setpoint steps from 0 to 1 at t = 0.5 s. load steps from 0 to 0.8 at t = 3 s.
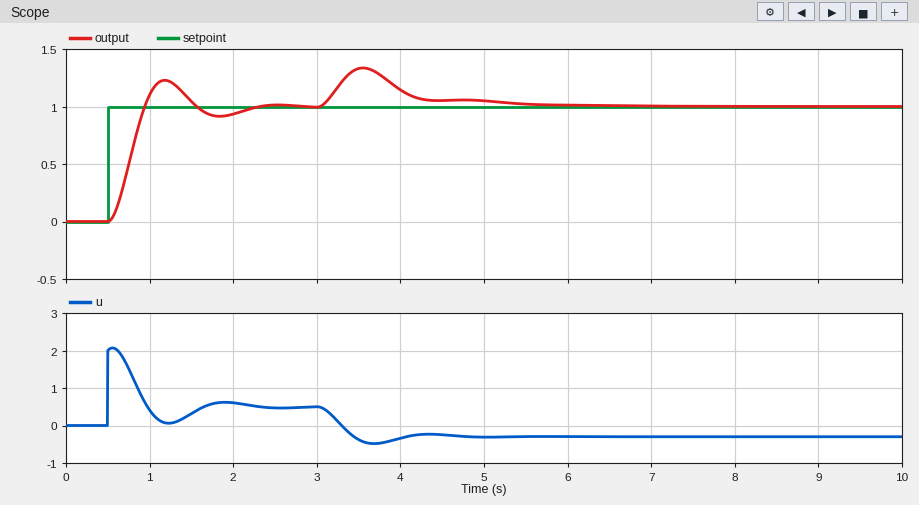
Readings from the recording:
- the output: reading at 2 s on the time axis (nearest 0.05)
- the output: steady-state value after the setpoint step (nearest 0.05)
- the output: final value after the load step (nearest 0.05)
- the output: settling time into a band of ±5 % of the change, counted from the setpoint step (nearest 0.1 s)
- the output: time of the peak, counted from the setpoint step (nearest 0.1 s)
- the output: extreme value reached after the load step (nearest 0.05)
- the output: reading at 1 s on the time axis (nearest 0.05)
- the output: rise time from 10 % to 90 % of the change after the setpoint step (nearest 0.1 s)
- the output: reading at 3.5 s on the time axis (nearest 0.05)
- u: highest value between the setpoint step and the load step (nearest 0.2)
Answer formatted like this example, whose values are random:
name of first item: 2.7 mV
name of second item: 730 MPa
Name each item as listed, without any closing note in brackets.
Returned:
the output: reading at 2 s on the time axis: 0.95
the output: steady-state value after the setpoint step: 1.00
the output: final value after the load step: 1.00
the output: settling time into a band of ±5 % of the change, counted from the setpoint step: 1.6 s
the output: time of the peak, counted from the setpoint step: 0.7 s
the output: extreme value reached after the load step: 1.35
the output: reading at 1 s on the time axis: 1.10
the output: rise time from 10 % to 90 % of the change after the setpoint step: 0.3 s
the output: reading at 3.5 s on the time axis: 1.35
u: highest value between the setpoint step and the load step: 2.0
